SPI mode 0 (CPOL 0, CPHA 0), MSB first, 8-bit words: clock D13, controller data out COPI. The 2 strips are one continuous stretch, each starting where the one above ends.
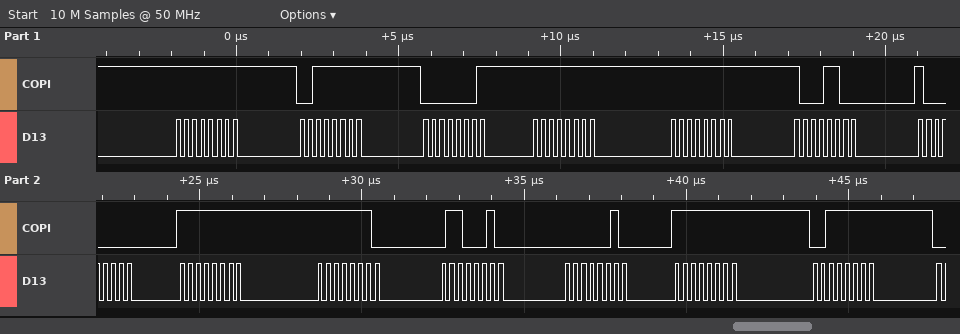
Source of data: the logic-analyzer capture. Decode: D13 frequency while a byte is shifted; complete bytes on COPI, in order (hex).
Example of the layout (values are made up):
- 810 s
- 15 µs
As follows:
- 4 MHz
- FF 3F 01 FF FF 8C 80 FF FE 62 02 FF 3F
